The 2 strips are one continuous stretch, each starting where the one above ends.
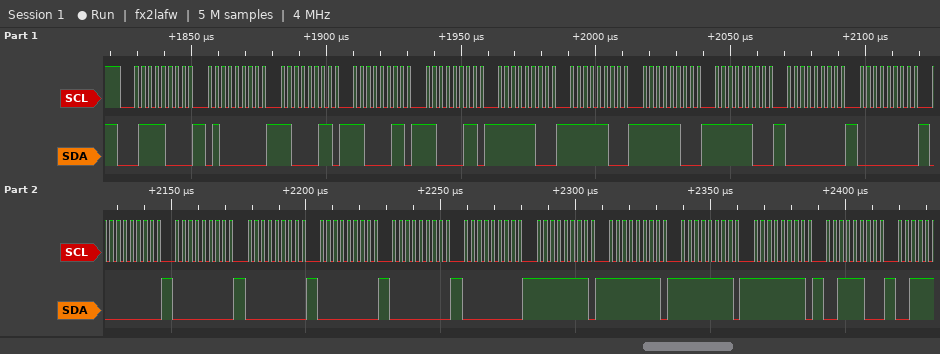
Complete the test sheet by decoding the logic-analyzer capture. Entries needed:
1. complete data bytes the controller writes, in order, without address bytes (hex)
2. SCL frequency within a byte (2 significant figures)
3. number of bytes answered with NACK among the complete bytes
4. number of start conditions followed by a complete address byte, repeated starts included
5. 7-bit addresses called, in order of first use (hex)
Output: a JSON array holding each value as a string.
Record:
["40 C3 C3 C3 FC FC FC FC 00 00 00 00 00 00 00 00 FF FF FF FF 3C", "400 kHz", "0", "1", "0x3C"]
